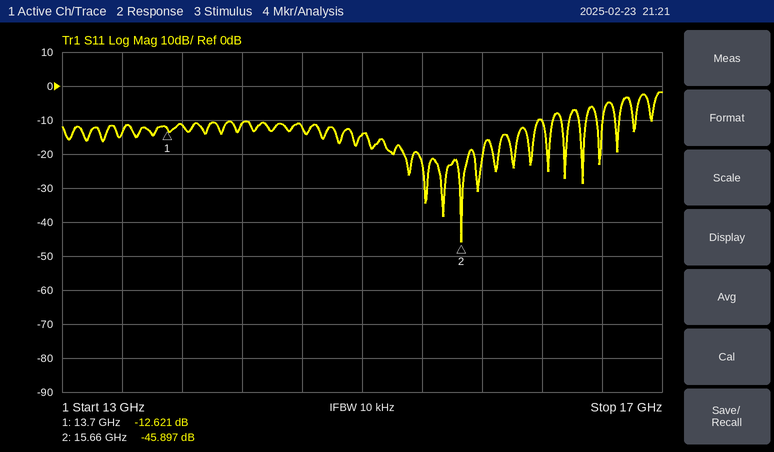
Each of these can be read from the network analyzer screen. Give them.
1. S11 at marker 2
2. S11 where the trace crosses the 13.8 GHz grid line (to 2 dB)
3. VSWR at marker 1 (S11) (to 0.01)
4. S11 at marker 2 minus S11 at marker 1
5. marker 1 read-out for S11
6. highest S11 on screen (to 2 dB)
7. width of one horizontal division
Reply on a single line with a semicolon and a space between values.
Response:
-45.897 dB; -12 dB; 1.61; -33.276 dB; -12.621 dB; -2 dB; 400 MHz
